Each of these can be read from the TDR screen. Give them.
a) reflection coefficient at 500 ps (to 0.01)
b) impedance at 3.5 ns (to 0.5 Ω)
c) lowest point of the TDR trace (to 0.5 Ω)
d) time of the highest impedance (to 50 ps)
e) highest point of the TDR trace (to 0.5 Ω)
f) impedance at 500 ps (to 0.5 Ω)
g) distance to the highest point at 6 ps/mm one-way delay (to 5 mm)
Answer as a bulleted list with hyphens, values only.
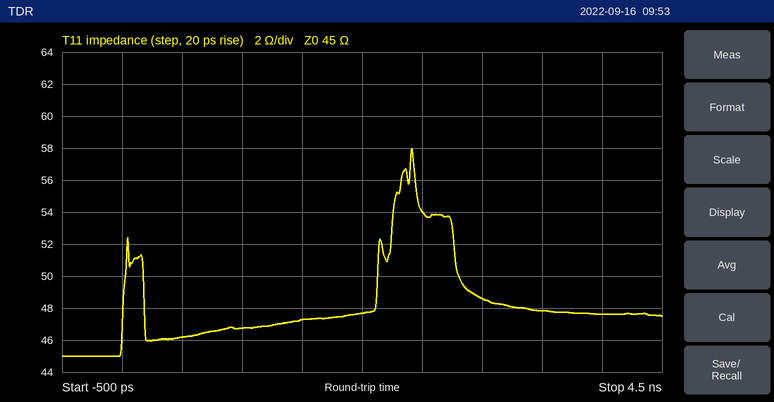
- +0.01
- 48.0 Ω
- 45.0 Ω
- 2.40 ns
- 58.0 Ω
- 46.0 Ω
- 200 mm
